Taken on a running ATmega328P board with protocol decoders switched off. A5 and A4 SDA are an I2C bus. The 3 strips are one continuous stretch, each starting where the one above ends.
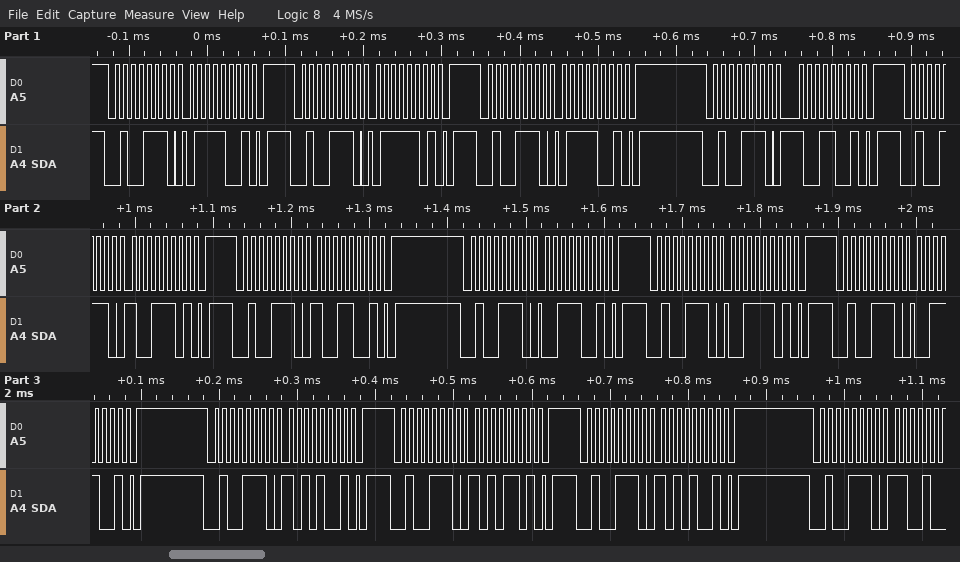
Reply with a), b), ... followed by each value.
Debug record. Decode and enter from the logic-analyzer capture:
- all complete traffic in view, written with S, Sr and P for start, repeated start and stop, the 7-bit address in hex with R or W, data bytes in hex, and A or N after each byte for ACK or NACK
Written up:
a) S 27W A 79 A P S 27W A 7D A P S 27W A 79 A P S 27W A 99 A P S 27W A 9D A P S 27W A 99 A P S 27W A 39 A P S 27W A 3D A P S 27W A 39 A P S 27W A A9 A P S 27W A AD A P S 27W A A9 A P S 27W A
